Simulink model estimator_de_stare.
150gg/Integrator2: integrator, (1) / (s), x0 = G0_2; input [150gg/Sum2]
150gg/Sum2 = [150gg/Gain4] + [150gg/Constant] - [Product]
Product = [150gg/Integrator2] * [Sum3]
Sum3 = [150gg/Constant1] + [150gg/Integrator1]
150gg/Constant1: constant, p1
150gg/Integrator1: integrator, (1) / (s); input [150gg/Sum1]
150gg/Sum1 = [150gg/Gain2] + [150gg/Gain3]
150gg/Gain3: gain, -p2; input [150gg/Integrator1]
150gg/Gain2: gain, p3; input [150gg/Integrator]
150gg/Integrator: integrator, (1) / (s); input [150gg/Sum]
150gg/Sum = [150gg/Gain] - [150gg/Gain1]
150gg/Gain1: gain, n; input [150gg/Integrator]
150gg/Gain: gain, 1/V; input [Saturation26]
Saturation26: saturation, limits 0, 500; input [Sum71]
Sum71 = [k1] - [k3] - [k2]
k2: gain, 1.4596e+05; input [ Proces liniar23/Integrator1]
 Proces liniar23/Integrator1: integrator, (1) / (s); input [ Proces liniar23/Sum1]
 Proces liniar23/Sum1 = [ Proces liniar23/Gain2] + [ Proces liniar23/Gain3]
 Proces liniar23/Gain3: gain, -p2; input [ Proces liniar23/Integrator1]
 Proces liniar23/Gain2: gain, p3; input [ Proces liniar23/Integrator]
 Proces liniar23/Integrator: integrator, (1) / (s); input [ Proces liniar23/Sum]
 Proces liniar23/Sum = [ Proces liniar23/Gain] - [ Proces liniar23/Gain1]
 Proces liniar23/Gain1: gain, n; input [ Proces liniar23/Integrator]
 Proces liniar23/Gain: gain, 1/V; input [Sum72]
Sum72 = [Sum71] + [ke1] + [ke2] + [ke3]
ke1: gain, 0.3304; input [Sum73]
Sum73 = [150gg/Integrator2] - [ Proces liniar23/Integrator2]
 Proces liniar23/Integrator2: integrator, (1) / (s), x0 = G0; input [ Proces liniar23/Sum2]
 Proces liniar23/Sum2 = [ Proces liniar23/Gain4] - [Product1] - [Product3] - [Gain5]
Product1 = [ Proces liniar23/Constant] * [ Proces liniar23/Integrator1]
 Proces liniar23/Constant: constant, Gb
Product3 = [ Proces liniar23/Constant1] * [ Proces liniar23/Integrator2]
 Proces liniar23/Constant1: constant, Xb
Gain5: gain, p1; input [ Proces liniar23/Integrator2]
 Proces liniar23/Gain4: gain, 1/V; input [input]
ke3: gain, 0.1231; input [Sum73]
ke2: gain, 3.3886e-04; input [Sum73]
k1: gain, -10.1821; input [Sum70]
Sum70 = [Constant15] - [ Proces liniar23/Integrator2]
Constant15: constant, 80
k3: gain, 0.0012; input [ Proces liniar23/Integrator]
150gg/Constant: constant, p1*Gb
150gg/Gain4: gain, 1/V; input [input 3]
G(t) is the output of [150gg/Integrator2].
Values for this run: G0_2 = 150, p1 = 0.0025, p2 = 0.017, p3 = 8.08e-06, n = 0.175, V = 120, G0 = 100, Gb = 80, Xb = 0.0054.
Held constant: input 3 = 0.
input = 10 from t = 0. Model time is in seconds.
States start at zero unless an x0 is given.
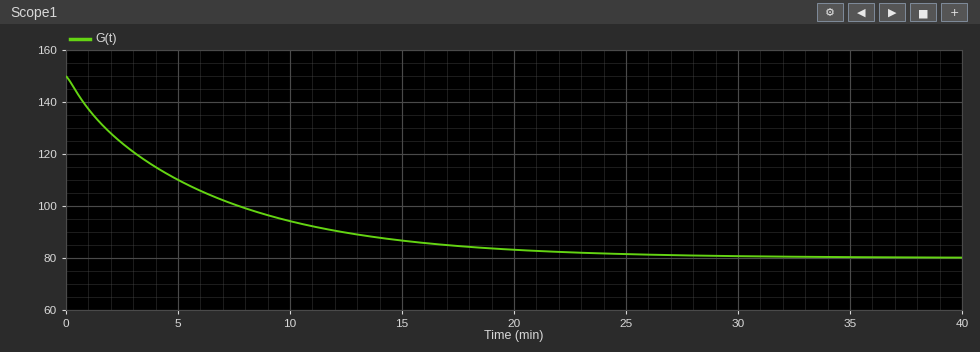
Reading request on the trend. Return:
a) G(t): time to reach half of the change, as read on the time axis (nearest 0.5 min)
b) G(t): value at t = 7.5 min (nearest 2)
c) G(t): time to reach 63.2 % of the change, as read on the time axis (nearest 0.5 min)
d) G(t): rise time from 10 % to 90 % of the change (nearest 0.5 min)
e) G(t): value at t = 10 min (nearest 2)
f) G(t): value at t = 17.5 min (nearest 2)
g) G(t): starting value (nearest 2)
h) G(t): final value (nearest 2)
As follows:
4.0 min
100
6.0 min
14.0 min
94
84
150
80
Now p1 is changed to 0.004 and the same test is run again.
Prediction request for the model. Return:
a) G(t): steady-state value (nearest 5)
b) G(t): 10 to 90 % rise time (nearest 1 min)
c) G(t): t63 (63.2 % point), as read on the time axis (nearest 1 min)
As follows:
80
9 min
4 min
